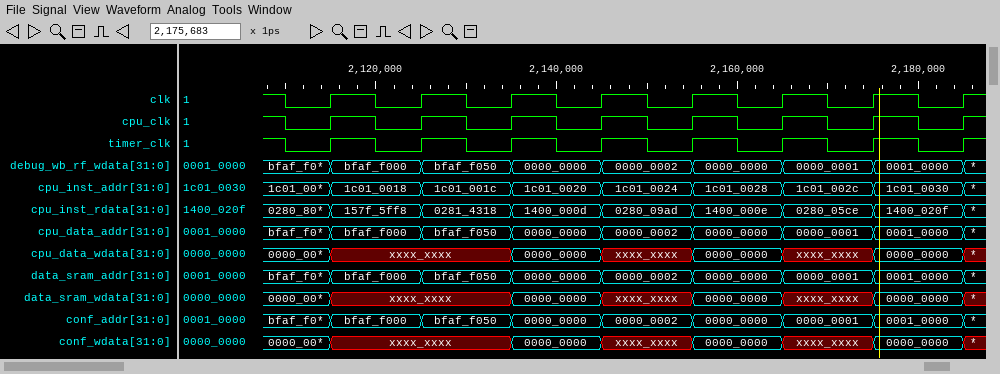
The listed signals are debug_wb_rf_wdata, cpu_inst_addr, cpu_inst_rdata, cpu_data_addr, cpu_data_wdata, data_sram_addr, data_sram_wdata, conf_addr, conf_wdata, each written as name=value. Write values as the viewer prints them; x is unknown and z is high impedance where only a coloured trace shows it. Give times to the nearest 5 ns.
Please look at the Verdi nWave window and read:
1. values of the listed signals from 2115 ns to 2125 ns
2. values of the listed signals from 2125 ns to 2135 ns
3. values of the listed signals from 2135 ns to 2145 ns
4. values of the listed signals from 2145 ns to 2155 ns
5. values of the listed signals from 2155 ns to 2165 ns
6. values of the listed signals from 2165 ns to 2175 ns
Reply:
debug_wb_rf_wdata=bfaf_f000, cpu_inst_addr=1c01_0018, cpu_inst_rdata=157f_5ff8, cpu_data_addr=bfaf_f000, cpu_data_wdata=xxxx_xxxx, data_sram_addr=bfaf_f000, data_sram_wdata=xxxx_xxxx, conf_addr=bfaf_f000, conf_wdata=xxxx_xxxx
debug_wb_rf_wdata=bfaf_f050, cpu_inst_addr=1c01_001c, cpu_inst_rdata=0281_4318, cpu_data_addr=bfaf_f050, cpu_data_wdata=xxxx_xxxx, data_sram_addr=bfaf_f050, data_sram_wdata=xxxx_xxxx, conf_addr=bfaf_f050, conf_wdata=xxxx_xxxx
debug_wb_rf_wdata=0000_0000, cpu_inst_addr=1c01_0020, cpu_inst_rdata=1400_000d, cpu_data_addr=0000_0000, cpu_data_wdata=0000_0000, data_sram_addr=0000_0000, data_sram_wdata=0000_0000, conf_addr=0000_0000, conf_wdata=0000_0000
debug_wb_rf_wdata=0000_0002, cpu_inst_addr=1c01_0024, cpu_inst_rdata=0280_09ad, cpu_data_addr=0000_0002, cpu_data_wdata=xxxx_xxxx, data_sram_addr=0000_0002, data_sram_wdata=xxxx_xxxx, conf_addr=0000_0002, conf_wdata=xxxx_xxxx
debug_wb_rf_wdata=0000_0000, cpu_inst_addr=1c01_0028, cpu_inst_rdata=1400_000e, cpu_data_addr=0000_0000, cpu_data_wdata=0000_0000, data_sram_addr=0000_0000, data_sram_wdata=0000_0000, conf_addr=0000_0000, conf_wdata=0000_0000
debug_wb_rf_wdata=0000_0001, cpu_inst_addr=1c01_002c, cpu_inst_rdata=0280_05ce, cpu_data_addr=0000_0001, cpu_data_wdata=xxxx_xxxx, data_sram_addr=0000_0001, data_sram_wdata=xxxx_xxxx, conf_addr=0000_0001, conf_wdata=xxxx_xxxx
